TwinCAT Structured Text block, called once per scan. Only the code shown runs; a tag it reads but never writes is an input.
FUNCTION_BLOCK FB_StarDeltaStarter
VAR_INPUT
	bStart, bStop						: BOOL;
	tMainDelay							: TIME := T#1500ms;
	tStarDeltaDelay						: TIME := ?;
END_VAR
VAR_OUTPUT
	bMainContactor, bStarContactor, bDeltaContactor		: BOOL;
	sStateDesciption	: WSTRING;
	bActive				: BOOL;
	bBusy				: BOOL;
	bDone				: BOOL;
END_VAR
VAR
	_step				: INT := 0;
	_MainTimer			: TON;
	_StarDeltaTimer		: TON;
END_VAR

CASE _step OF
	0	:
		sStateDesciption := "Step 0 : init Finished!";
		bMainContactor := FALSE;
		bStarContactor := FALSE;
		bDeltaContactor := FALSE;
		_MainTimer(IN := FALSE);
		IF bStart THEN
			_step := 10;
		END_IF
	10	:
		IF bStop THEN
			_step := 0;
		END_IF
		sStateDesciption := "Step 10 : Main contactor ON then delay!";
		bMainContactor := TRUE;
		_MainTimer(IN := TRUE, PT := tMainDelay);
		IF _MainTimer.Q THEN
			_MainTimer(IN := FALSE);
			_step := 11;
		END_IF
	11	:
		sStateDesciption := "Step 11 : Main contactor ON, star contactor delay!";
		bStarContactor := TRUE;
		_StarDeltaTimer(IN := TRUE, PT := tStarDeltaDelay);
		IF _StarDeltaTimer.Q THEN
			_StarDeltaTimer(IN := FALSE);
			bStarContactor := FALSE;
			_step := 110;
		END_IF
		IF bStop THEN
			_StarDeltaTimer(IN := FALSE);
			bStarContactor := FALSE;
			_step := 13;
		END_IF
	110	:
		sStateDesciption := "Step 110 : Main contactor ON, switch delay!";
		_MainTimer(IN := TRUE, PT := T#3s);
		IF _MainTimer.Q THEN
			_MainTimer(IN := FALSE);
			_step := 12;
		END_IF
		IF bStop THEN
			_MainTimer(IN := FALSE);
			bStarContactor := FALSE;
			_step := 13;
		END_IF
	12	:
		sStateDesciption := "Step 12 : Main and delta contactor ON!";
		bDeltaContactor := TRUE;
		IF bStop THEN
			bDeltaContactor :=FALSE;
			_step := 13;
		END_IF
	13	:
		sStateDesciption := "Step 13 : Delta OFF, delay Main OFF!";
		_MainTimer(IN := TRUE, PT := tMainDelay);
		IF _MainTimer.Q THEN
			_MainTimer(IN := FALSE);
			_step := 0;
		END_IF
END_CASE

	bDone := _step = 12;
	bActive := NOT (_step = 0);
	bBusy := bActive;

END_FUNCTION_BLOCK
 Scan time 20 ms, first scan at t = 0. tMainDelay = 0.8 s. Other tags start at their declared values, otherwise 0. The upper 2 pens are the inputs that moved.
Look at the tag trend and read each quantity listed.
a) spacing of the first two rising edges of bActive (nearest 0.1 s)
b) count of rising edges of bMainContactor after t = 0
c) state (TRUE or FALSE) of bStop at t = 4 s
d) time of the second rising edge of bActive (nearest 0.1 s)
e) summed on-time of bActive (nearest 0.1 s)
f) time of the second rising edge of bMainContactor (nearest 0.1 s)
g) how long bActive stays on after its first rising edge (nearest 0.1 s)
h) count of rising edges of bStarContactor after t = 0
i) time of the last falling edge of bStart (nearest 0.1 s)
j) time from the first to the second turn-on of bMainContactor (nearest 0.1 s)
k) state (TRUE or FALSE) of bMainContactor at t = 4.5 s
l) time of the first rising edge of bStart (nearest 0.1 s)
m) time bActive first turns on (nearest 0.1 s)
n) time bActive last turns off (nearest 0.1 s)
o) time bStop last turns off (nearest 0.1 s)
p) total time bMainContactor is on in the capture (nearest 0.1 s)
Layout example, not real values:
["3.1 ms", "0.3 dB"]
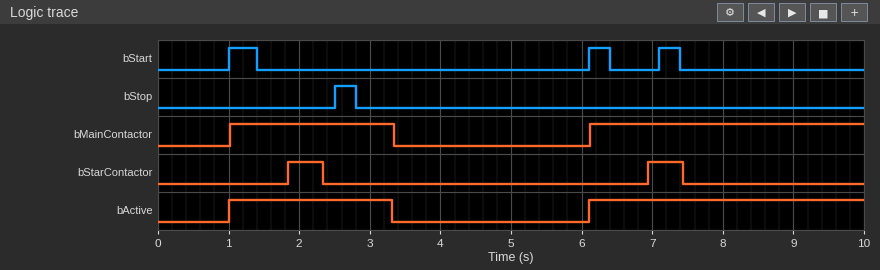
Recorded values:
["5.1 s", "2", "FALSE", "6.1 s", "6.2 s", "6.1 s", "2.3 s", "2", "7.4 s", "5.1 s", "FALSE", "1.0 s", "1.0 s", "3.3 s", "2.8 s", "6.2 s"]
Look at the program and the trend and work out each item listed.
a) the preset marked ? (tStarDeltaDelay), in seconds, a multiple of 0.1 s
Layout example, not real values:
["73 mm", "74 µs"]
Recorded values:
["0.5 s"]
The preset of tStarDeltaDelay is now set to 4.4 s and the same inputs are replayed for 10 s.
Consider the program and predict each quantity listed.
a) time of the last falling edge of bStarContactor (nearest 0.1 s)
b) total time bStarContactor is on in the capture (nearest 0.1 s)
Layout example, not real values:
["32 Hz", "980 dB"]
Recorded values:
["2.5 s", "3.7 s"]
